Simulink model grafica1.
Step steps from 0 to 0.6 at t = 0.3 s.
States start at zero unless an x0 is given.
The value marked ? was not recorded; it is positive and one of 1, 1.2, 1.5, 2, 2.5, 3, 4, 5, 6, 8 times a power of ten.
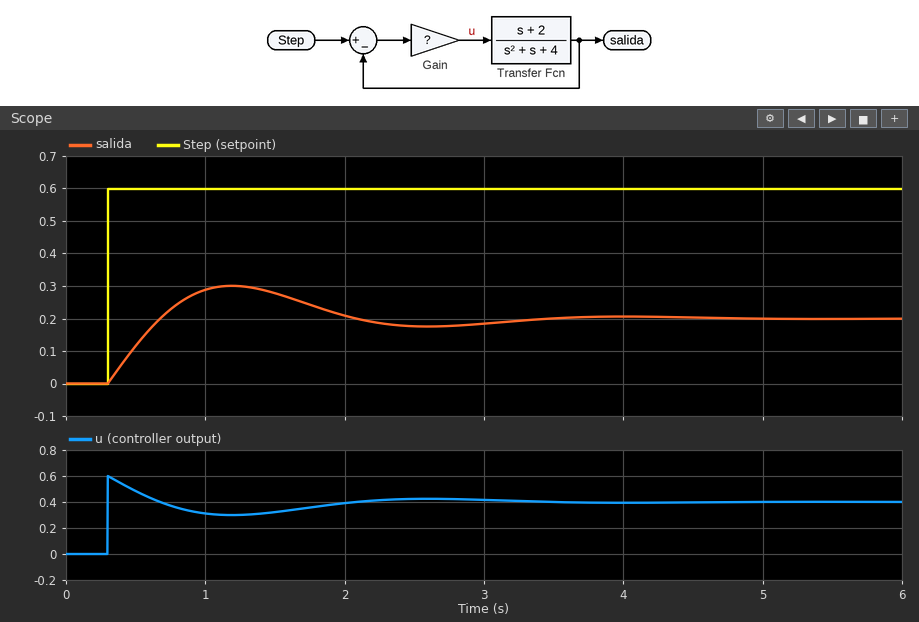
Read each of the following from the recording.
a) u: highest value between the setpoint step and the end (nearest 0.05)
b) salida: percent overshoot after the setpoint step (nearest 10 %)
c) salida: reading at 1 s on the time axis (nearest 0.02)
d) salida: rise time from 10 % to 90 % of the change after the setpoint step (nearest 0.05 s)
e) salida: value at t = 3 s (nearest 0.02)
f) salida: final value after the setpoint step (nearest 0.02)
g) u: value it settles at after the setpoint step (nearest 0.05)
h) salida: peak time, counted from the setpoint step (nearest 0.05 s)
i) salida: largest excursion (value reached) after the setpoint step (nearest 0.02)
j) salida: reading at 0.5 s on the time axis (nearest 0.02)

0.60
50 %
0.28
0.30 s
0.18
0.20
0.40
0.90 s
0.30
0.12
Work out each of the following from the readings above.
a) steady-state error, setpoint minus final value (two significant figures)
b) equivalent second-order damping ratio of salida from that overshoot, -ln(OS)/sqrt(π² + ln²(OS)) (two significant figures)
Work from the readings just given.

0.40
0.22
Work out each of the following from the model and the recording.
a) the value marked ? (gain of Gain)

1
